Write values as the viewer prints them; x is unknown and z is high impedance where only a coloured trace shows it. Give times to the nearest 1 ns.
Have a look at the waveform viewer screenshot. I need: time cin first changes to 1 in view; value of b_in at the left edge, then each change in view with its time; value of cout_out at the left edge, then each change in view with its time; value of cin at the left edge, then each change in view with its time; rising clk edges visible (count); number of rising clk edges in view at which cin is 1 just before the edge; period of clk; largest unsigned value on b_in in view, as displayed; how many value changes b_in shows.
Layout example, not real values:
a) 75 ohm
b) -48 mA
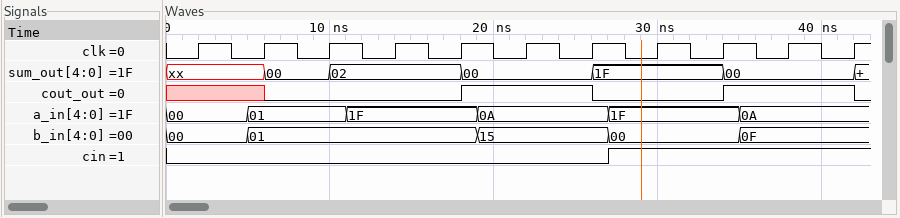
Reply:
a) 27 ns
b) 00, 01 at 5 ns, 15 at 19 ns, 00 at 27 ns, 0F at 35 ns
c) x, 0 at 6 ns, 1 at 18 ns, 0 at 26 ns, 1 at 34 ns, 0 at 42 ns
d) 0, 1 at 27 ns
e) 11
f) 4
g) 4 ns
h) 15
i) 4
